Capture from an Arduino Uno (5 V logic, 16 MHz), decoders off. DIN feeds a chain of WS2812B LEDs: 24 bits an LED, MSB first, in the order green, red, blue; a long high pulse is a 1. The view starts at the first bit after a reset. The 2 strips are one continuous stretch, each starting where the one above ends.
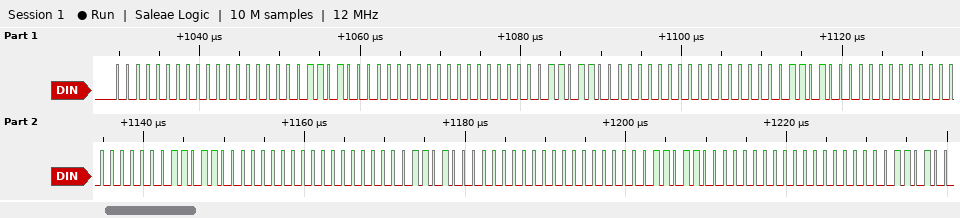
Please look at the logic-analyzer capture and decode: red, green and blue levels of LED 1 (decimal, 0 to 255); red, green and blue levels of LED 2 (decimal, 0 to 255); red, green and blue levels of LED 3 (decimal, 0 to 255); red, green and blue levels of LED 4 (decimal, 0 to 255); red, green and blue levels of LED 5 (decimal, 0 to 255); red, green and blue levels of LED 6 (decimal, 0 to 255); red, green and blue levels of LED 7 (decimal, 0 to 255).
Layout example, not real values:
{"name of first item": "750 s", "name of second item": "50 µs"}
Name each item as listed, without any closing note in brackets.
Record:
{"red, green and blue levels of LED 1": "0, 0, 26", "red, green and blue levels of LED 2": "0, 0, 27", "red, green and blue levels of LED 3": "0, 0, 26", "red, green and blue levels of LED 4": "0, 0, 27", "red, green and blue levels of LED 5": "0, 0, 26", "red, green and blue levels of LED 6": "0, 0, 27", "red, green and blue levels of LED 7": "0, 0, 26"}
